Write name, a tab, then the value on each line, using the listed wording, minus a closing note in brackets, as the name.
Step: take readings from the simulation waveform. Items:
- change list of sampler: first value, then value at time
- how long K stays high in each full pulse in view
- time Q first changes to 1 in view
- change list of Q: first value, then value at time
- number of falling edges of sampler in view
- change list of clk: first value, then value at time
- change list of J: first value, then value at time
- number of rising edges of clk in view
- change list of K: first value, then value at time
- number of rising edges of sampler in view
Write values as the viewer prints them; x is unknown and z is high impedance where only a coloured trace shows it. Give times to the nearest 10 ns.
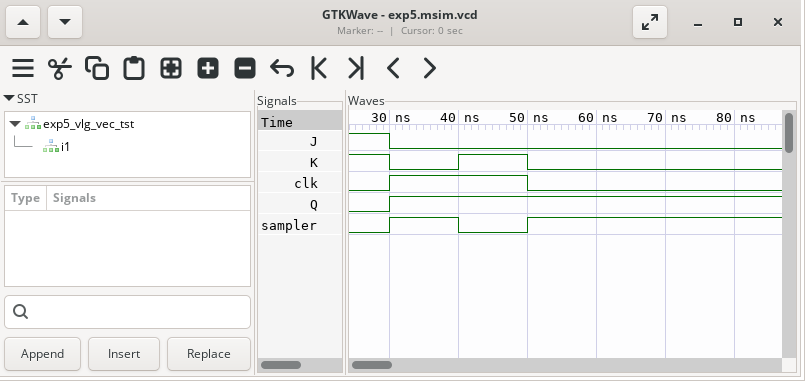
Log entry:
change list of sampler: first value, then value at time	0, 1 at 30 ns, 0 at 40 ns, 1 at 50 ns
how long K stays high in each full pulse in view	10 ns
time Q first changes to 1 in view	30 ns
change list of Q: first value, then value at time	0, 1 at 30 ns
number of falling edges of sampler in view	1
change list of clk: first value, then value at time	0, 1 at 30 ns, 0 at 50 ns
change list of J: first value, then value at time	1, 0 at 30 ns
number of rising edges of clk in view	1
change list of K: first value, then value at time	1, 0 at 30 ns, 1 at 40 ns, 0 at 50 ns
number of rising edges of sampler in view	2
